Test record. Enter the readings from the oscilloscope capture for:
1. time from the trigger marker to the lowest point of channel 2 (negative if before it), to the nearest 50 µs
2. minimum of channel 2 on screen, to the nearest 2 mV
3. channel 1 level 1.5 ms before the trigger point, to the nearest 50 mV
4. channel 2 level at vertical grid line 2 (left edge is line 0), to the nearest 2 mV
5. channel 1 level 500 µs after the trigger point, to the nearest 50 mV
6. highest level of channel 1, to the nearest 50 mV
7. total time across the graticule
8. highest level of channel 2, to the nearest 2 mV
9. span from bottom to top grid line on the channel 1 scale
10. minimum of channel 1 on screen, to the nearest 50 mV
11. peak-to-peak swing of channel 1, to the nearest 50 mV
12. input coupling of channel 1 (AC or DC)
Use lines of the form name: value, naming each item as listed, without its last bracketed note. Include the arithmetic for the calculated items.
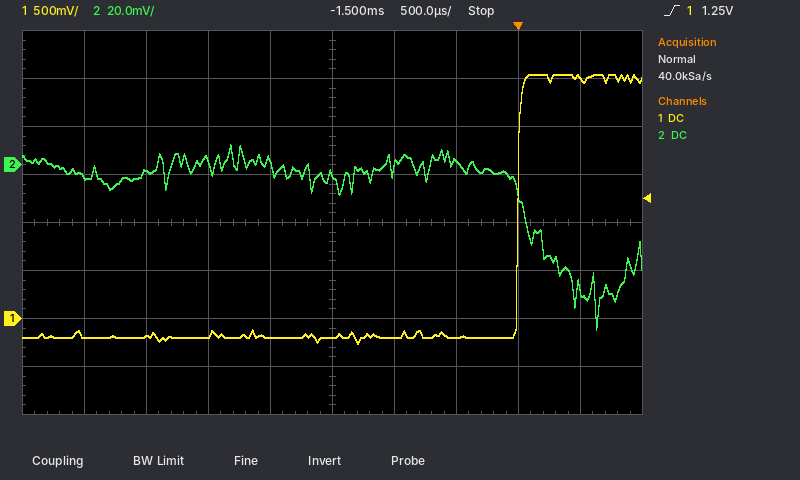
time from the trigger marker to the lowest point of channel 2 (negative if before it), to the nearest 50 µs: +650 µs
minimum of channel 2 on screen, to the nearest 2 mV: -68 mV
channel 1 level 1.5 ms before the trigger point, to the nearest 50 mV: -200 mV
channel 2 level at vertical grid line 2 (left edge is line 0), to the nearest 2 mV: -2 mV
channel 1 level 500 µs after the trigger point, to the nearest 50 mV: 2.50 V
highest level of channel 1, to the nearest 50 mV: 2.55 V
total time across the graticule: 5 ms
highest level of channel 2, to the nearest 2 mV: 8 mV
span from bottom to top grid line on the channel 1 scale: 4 V
minimum of channel 1 on screen, to the nearest 50 mV: -250 mV
peak-to-peak swing of channel 1, to the nearest 50 mV: 2.55 V − (-250 mV) = 2.80 V
input coupling of channel 1: DC
